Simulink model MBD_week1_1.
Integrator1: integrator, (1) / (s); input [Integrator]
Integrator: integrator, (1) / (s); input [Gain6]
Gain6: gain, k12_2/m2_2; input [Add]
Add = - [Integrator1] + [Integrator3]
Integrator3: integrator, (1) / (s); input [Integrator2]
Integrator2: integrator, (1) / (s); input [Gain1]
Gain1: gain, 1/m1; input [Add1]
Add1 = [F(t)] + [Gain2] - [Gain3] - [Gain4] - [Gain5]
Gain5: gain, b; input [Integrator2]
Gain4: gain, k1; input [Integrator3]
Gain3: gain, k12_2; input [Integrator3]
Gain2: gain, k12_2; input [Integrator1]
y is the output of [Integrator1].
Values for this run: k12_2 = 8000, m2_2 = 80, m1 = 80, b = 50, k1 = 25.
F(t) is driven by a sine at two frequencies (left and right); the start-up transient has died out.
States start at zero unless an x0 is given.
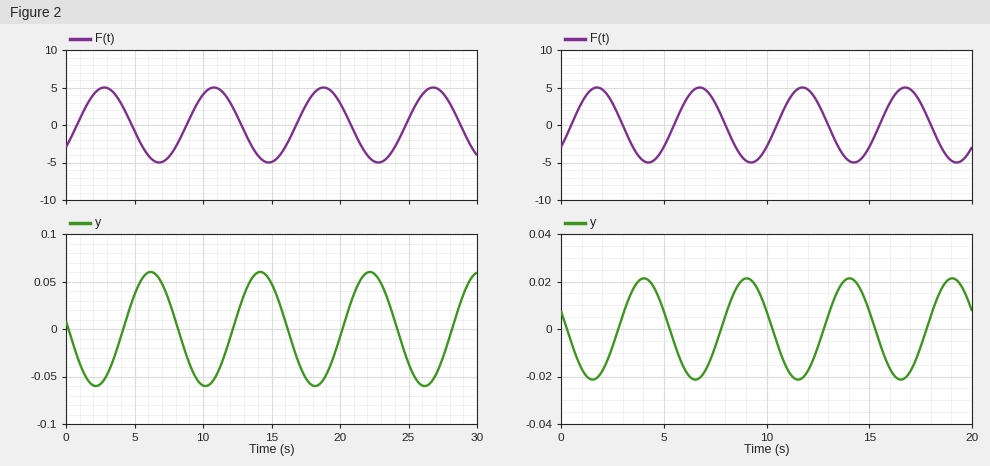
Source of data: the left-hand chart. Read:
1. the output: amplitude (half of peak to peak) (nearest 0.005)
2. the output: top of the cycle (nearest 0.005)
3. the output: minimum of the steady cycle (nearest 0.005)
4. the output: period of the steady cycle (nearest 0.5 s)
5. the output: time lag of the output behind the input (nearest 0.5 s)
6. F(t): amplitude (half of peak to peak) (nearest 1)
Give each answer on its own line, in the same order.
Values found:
0.060
0.060
-0.060
8.0 s
3.5 s
5
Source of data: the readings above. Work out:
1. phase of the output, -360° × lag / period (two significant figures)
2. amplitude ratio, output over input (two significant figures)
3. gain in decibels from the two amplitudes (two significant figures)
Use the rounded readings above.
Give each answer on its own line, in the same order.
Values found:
-160°
0.012
-38 dB
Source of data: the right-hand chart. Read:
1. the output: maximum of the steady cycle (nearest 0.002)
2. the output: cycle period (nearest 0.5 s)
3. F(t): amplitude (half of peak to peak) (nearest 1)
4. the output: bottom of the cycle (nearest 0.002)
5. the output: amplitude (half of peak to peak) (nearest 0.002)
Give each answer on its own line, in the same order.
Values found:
0.022
5.0 s
5
-0.022
0.022
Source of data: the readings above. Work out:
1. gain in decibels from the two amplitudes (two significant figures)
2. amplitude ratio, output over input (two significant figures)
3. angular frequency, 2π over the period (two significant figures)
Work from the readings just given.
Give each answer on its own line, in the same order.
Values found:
-47 dB
0.0044
1.3 rad/s
